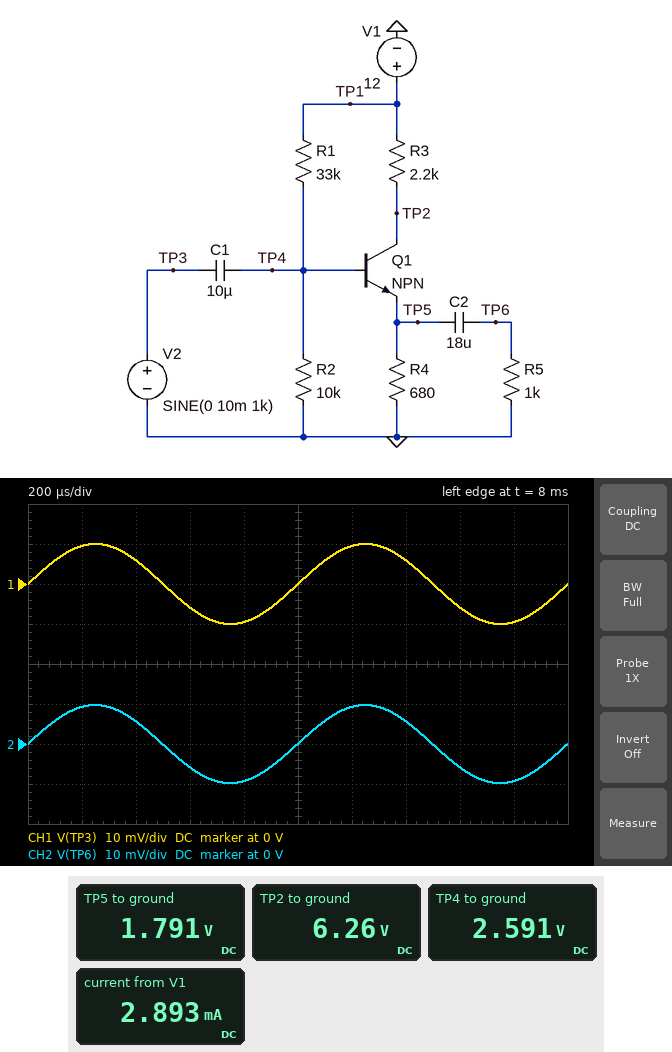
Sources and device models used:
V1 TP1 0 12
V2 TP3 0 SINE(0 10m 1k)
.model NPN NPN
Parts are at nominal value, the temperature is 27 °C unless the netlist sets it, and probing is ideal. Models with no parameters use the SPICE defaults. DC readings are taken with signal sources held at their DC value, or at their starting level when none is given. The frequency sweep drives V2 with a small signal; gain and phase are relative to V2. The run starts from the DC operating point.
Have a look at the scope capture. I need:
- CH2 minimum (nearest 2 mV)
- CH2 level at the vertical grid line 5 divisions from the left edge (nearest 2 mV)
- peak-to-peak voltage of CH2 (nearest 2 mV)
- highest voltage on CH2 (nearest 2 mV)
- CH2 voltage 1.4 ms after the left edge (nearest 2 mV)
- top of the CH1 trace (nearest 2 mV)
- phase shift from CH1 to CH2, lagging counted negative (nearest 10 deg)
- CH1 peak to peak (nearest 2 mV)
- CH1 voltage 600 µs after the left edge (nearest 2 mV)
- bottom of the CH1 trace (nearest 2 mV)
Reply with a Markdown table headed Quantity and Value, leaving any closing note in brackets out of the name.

| Quantity | Value |
|---|---|
| CH2 minimum | -10 mV |
| CH2 level at the vertical grid line 5 divisions from the left edge | 0 V |
| peak-to-peak voltage of CH2 | 20 mV |
| highest voltage on CH2 | 10 mV |
| CH2 voltage 1.4 ms after the left edge | 6 mV |
| top of the CH1 trace | 10 mV |
| phase shift from CH1 to CH2, lagging counted negative | 0 deg |
| CH1 peak to peak | 20 mV |
| CH1 voltage 600 µs after the left edge | -6 mV |
| bottom of the CH1 trace | -10 mV |
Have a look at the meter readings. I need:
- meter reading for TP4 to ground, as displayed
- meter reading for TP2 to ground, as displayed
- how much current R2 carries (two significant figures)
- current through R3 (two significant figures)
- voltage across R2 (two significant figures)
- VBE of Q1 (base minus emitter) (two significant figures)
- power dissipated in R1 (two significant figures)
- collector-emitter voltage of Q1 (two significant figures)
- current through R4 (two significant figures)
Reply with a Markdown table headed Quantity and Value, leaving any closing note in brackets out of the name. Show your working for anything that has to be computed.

| Quantity | Value |
|---|---|
| meter reading for TP4 to ground, as displayed | 2.591 V |
| meter reading for TP2 to ground, as displayed | 6.26 V |
| how much current R2 carries | (2.591 V) / 10 kΩ = 260 µA |
| current through R3 | (12 V - 6.26 V) / 2.2 kΩ = 2.6 mA |
| voltage across R2 | 2.591 V = 2.6 V |
| VBE of Q1 (base minus emitter) | 2.591 V - 1.791 V = 800 mV |
| power dissipated in R1 | (12 V - 2.591 V)^2 / 33 kΩ = 2.7 mW |
| collector-emitter voltage of Q1 | 6.26 V - 1.791 V = 4.5 V |
| current through R4 | (1.791 V) / 680 Ω = 2.6 mA |
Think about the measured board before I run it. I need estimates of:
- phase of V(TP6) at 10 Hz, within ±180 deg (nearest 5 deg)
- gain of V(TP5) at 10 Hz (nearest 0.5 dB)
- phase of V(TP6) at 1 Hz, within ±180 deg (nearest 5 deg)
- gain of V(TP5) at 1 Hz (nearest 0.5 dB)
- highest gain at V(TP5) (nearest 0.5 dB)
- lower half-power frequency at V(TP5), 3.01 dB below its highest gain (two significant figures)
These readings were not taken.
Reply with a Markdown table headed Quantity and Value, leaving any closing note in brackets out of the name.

| Quantity | Value |
|---|---|
| phase of V(TP6) at 10 Hz, within ±180 deg | 55 deg |
| gain of V(TP5) at 10 Hz | -0.5 dB |
| phase of V(TP6) at 1 Hz, within ±180 deg | 150 deg |
| gain of V(TP5) at 1 Hz | -8.0 dB |
| highest gain at V(TP5) | 0 dB |
| lower half-power frequency at V(TP5), 3.01 dB below its highest gain | 2.3 Hz |
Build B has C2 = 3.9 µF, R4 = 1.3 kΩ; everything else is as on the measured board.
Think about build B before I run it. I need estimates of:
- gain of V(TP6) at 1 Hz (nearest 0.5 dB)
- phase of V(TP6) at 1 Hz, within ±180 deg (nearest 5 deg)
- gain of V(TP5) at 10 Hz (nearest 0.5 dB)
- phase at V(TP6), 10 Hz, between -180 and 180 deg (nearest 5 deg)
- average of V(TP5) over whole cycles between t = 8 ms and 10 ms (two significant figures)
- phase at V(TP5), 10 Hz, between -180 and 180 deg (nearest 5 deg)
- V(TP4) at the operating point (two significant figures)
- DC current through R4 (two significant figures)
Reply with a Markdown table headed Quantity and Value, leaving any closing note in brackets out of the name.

| Quantity | Value |
|---|---|
| gain of V(TP6) at 1 Hz | -40.0 dB |
| phase of V(TP6) at 1 Hz, within ±180 deg | 155 deg |
| gain of V(TP5) at 10 Hz | -0.5 dB |
| phase at V(TP6), 10 Hz, between -180 and 180 deg | 90 deg |
| average of V(TP5) over whole cycles between t = 8 ms and 10 ms | 1.9 V |
| phase at V(TP5), 10 Hz, between -180 and 180 deg | 10 deg |
| V(TP4) at the operating point | 2.7 V |
| DC current through R4 | 1.5 mA |
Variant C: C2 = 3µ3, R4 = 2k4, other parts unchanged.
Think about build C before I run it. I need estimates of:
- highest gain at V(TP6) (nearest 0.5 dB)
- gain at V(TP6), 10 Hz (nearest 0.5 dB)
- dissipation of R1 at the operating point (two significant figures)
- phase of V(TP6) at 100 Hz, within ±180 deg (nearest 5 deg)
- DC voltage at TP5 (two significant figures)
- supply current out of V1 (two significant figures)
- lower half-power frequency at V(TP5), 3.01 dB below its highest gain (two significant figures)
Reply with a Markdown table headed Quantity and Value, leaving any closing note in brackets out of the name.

| Quantity | Value |
|---|---|
| highest gain at V(TP6) | -0.5 dB |
| gain at V(TP6), 10 Hz | -14.0 dB |
| dissipation of R1 at the operating point | 2.6 mW |
| phase of V(TP6) at 100 Hz, within ±180 deg | 25 deg |
| DC voltage at TP5 | 2.0 V |
| supply current out of V1 | 1.1 mA |
| lower half-power frequency at V(TP5), 3.01 dB below its highest gain | 2.1 Hz |
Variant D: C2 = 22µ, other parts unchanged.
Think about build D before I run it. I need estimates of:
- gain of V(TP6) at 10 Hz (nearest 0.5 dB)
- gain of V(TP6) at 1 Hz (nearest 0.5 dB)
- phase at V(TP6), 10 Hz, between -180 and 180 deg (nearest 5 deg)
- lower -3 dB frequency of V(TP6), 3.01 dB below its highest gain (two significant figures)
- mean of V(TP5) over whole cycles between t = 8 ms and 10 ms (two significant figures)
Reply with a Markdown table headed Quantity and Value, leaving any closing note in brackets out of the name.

| Quantity | Value |
|---|---|
| gain of V(TP6) at 10 Hz | -2.5 dB |
| gain of V(TP6) at 1 Hz | -25.5 dB |
| phase at V(TP6), 10 Hz, between -180 and 180 deg | 50 deg |
| lower -3 dB frequency of V(TP6), 3.01 dB below its highest gain | 8.0 Hz |
| mean of V(TP5) over whole cycles between t = 8 ms and 10 ms | 1.8 V |
